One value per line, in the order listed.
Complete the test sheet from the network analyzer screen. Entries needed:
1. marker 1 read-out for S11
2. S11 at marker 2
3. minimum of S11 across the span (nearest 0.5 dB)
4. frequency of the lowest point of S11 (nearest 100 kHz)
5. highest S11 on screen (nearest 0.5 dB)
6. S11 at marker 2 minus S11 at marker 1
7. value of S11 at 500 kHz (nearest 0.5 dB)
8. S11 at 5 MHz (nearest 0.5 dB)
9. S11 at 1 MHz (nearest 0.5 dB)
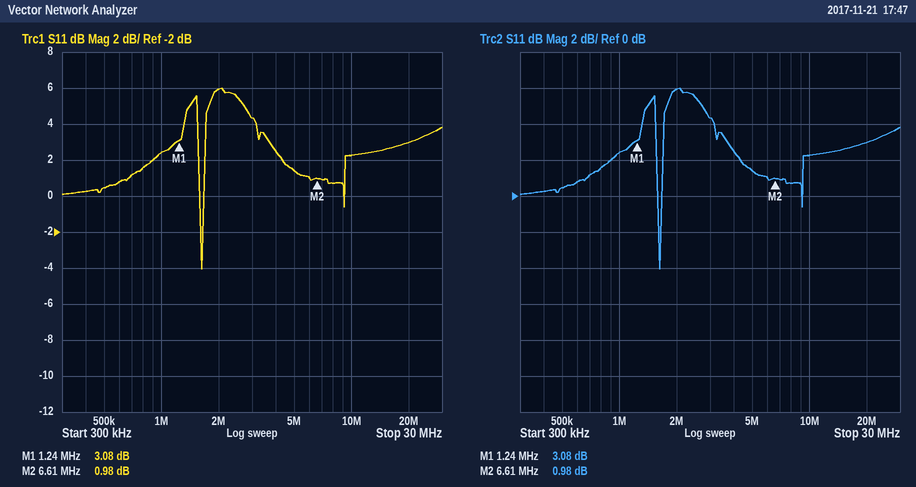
3.08 dB
0.98 dB
-4.0 dB
1.6 MHz
6.0 dB
-2.10 dB
0.5 dB
1.5 dB
2.5 dB
